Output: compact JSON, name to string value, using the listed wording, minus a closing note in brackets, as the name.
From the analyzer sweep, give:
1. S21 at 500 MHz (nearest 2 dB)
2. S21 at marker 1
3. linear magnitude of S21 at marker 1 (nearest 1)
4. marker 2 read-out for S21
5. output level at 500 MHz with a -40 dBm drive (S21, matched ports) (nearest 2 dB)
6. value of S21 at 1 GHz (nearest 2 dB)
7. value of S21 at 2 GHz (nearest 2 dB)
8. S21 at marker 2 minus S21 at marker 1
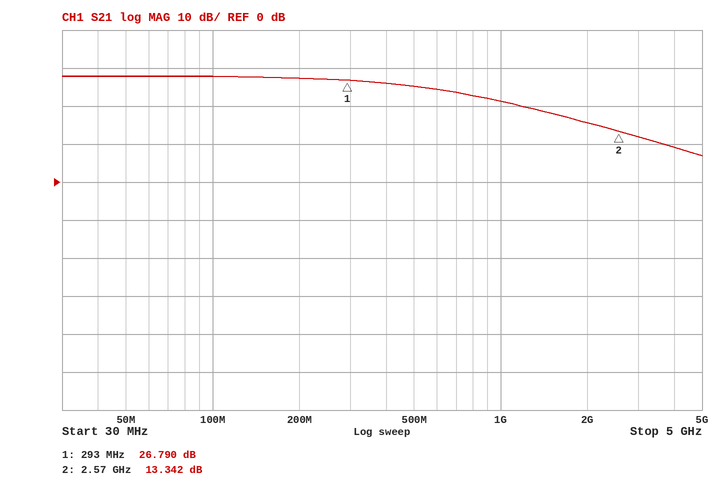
{"S21 at 500 MHz": "26 dB", "S21 at marker 1": "26.790 dB", "linear magnitude of S21 at marker 1": "22", "marker 2 read-out for S21": "13.342 dB", "output level at 500 MHz with a -40 dBm drive (S21, matched ports)": "-14 dBm", "value of S21 at 1 GHz": "22 dB", "value of S21 at 2 GHz": "16 dB", "S21 at marker 2 minus S21 at marker 1": "-13.448 dB"}
